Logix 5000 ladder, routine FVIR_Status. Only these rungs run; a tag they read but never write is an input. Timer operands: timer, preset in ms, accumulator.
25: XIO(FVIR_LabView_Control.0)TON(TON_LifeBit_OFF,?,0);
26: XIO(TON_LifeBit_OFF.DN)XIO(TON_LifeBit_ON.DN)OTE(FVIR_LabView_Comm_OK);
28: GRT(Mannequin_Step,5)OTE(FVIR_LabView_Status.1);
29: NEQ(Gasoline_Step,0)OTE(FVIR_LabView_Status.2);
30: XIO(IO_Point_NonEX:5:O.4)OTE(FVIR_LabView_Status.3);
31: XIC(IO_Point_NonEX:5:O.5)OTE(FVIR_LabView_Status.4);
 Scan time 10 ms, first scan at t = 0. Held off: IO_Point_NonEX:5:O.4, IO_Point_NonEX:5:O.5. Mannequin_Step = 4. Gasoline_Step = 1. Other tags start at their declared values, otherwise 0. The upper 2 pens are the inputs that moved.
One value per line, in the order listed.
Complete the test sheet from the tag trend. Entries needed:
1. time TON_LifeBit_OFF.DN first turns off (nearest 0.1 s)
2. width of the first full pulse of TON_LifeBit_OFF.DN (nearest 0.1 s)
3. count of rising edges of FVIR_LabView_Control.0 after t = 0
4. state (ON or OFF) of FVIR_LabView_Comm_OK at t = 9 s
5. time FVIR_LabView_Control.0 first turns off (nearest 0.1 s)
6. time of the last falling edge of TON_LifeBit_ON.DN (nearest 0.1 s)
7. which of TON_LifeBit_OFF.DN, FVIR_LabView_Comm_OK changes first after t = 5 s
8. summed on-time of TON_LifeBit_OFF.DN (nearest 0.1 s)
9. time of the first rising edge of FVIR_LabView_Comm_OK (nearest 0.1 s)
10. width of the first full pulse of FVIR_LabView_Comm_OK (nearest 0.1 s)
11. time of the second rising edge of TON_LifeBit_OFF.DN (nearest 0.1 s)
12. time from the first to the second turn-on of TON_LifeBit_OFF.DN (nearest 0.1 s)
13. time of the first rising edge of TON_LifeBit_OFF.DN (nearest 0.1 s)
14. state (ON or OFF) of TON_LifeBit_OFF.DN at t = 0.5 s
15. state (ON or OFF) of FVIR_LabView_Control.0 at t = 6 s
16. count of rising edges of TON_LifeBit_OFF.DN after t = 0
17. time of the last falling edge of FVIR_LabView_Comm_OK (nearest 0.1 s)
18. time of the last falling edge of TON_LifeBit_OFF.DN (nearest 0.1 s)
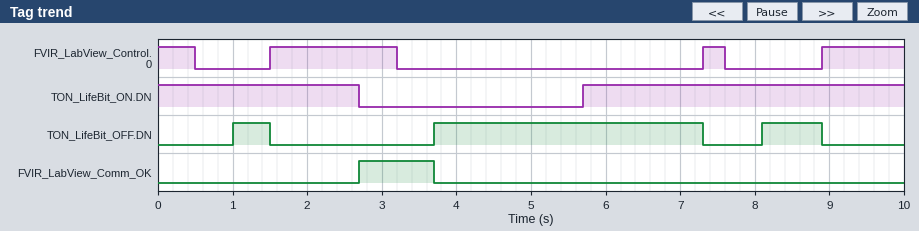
1.5 s
0.5 s
3
OFF
0.5 s
2.7 s
TON_LifeBit_OFF.DN
4.9 s
2.7 s
1.0 s
3.7 s
2.7 s
1.0 s
OFF
OFF
3
3.7 s
8.9 s
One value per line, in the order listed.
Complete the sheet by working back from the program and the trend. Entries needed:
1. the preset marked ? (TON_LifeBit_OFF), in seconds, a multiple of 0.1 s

0.5 s
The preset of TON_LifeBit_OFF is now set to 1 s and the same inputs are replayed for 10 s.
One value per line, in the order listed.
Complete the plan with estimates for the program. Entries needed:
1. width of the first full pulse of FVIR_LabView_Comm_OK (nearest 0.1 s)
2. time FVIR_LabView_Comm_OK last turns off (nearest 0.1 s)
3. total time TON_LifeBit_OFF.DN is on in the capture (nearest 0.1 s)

1.5 s
4.2 s
3.4 s
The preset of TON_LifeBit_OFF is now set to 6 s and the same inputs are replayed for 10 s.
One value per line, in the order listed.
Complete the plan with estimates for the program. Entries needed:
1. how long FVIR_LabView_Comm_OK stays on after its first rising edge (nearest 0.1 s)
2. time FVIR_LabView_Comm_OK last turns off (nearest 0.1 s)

3.0 s
5.7 s
